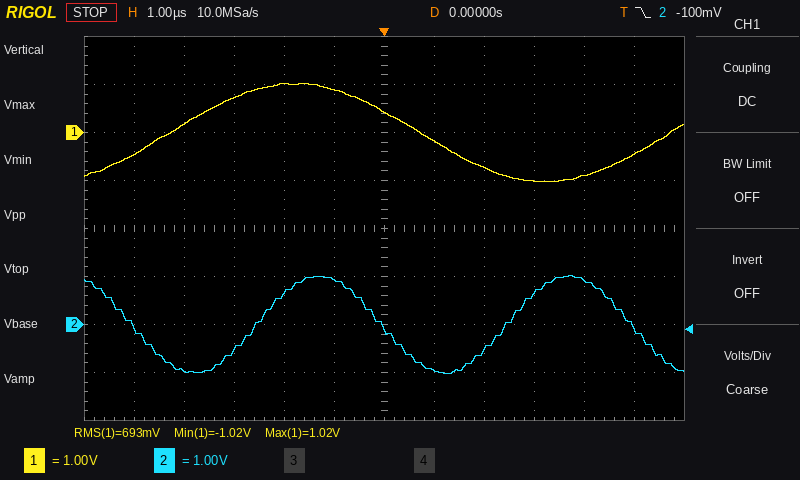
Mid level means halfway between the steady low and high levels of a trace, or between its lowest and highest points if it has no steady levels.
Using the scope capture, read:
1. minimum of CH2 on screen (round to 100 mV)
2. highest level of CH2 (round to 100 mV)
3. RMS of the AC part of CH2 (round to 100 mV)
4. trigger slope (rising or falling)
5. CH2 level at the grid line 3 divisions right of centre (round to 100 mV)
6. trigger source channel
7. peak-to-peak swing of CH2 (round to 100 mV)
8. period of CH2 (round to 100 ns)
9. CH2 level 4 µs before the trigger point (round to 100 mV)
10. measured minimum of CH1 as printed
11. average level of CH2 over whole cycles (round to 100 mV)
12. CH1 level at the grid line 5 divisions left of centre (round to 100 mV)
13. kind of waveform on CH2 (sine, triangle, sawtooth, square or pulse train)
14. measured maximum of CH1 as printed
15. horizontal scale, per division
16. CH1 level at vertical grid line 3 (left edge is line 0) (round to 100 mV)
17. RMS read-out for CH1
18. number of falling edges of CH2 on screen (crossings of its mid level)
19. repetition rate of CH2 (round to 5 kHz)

-1.0 V
1.0 V
700 mV
falling
600 mV
CH2
2.0 V
5.0 µs
-1.0 V
-1.02 V
0.0 V
-500 mV
sine
1.02 V
1 µs
700 mV
693 mV
3
200 kHz
